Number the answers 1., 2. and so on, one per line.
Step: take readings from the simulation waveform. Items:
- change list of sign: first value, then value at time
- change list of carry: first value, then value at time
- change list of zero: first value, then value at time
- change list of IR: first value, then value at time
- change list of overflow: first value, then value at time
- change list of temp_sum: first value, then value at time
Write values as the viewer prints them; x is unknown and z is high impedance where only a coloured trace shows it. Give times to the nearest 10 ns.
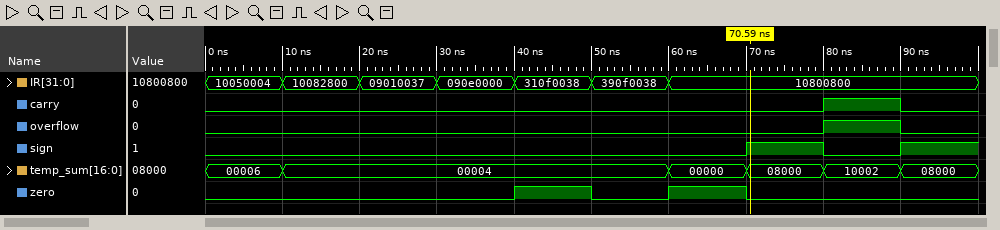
1. 0, 1 at 70 ns, 0 at 80 ns, 1 at 90 ns
2. 0, 1 at 80 ns, 0 at 90 ns
3. 0, 1 at 40 ns, 0 at 50 ns, 1 at 60 ns, 0 at 70 ns
4. 10050004, 10082800 at 10 ns, 09010037 at 20 ns, 090e0000 at 30 ns, 310f0038 at 40 ns, 390f0038 at 50 ns, 10800800 at 60 ns
5. 0, 1 at 80 ns, 0 at 90 ns
6. 00006, 00004 at 10 ns, 00000 at 60 ns, 08000 at 70 ns, 10002 at 80 ns, 08000 at 90 ns
